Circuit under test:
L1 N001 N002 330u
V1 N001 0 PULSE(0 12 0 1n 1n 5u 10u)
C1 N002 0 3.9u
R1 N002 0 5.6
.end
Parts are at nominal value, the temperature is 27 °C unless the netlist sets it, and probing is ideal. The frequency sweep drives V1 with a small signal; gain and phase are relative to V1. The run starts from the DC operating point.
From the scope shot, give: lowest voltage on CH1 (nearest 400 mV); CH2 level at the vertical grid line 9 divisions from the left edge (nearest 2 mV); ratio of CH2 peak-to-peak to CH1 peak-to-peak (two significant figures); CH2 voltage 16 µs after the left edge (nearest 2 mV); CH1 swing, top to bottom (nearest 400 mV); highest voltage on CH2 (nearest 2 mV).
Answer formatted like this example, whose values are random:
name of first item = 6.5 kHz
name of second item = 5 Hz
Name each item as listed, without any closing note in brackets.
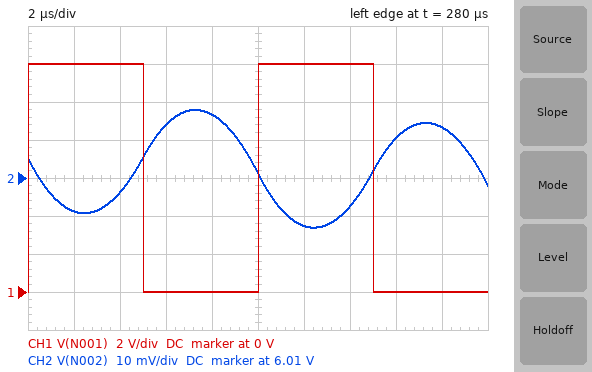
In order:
lowest voltage on CH1 = 0 V
CH2 level at the vertical grid line 9 divisions from the left edge = 6.024 V
ratio of CH2 peak-to-peak to CH1 peak-to-peak = 0.0026
CH2 voltage 16 µs after the left edge = 6.020 V
CH1 swing, top to bottom = 12.0 V
highest voltage on CH2 = 6.028 V
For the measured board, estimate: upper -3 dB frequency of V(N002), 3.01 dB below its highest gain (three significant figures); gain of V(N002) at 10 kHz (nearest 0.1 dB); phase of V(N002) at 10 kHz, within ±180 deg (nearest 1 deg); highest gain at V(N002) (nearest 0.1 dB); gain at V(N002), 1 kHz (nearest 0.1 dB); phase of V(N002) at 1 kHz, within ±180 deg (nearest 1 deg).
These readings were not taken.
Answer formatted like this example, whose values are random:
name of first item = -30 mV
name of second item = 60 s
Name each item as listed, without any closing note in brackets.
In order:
upper -3 dB frequency of V(N002), 3.01 dB below its highest gain = 3.74 kHz
gain of V(N002) at 10 kHz = -14.8 dB
phase of V(N002) at 10 kHz, within ±180 deg = -138 deg
highest gain at V(N002) = 0 dB
gain at V(N002), 1 kHz = -0.2 dB
phase of V(N002) at 1 kHz, within ±180 deg = -21 deg
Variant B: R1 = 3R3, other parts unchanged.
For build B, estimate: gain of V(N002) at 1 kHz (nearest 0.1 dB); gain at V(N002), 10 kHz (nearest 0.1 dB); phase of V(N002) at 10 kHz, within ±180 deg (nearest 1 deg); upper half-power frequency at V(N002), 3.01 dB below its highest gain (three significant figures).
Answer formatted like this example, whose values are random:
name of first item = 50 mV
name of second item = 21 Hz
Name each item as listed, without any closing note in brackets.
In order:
gain of V(N002) at 1 kHz = -1.1 dB
gain at V(N002), 10 kHz = -17.5 dB
phase of V(N002) at 10 kHz, within ±180 deg = -123 deg
upper half-power frequency at V(N002), 3.01 dB below its highest gain = 1.82 kHz
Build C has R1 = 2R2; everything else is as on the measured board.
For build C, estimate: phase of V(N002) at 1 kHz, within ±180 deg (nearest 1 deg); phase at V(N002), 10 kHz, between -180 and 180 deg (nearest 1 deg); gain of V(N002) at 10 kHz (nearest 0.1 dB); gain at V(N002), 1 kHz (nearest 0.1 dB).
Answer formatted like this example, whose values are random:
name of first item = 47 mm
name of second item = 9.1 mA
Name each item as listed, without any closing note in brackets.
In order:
phase of V(N002) at 1 kHz, within ±180 deg = -45 deg
phase at V(N002), 10 kHz, between -180 and 180 deg = -113 deg
gain of V(N002) at 10 kHz = -20.2 dB
gain at V(N002), 1 kHz = -2.5 dB
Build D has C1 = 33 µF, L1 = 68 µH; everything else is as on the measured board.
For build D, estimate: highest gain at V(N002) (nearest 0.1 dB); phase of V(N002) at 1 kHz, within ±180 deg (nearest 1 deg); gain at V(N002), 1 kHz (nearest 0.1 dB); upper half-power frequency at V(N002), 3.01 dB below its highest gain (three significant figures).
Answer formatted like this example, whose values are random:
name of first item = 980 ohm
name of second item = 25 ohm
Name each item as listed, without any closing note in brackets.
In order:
highest gain at V(N002) = 11.9 dB
phase of V(N002) at 1 kHz, within ±180 deg = -5 deg
gain at V(N002), 1 kHz = 0.8 dB
upper half-power frequency at V(N002), 3.01 dB below its highest gain = 3.71 kHz
